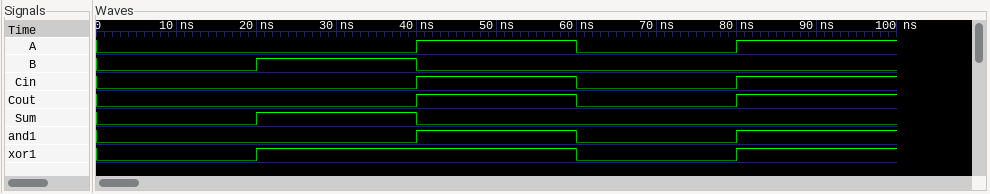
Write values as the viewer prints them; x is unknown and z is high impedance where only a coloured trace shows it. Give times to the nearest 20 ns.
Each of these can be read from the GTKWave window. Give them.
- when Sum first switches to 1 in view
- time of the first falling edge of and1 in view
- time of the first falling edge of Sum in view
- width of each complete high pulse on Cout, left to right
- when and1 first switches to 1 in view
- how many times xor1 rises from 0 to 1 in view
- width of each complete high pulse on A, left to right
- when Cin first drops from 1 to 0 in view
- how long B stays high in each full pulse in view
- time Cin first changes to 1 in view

20 ns
60 ns
40 ns
20 ns
40 ns
2
20 ns
60 ns
20 ns
40 ns
